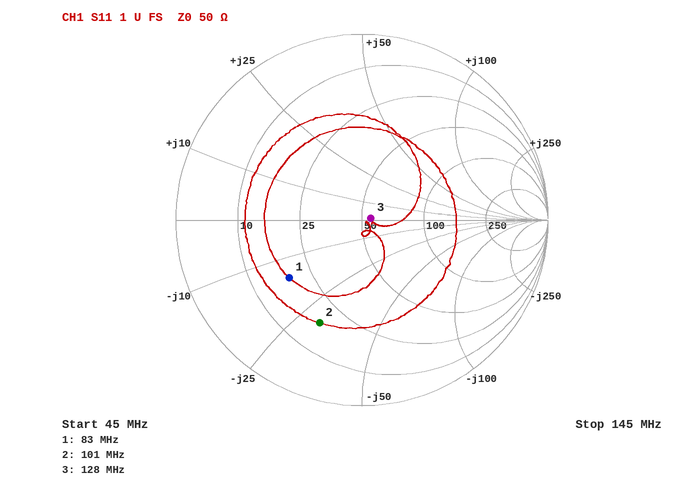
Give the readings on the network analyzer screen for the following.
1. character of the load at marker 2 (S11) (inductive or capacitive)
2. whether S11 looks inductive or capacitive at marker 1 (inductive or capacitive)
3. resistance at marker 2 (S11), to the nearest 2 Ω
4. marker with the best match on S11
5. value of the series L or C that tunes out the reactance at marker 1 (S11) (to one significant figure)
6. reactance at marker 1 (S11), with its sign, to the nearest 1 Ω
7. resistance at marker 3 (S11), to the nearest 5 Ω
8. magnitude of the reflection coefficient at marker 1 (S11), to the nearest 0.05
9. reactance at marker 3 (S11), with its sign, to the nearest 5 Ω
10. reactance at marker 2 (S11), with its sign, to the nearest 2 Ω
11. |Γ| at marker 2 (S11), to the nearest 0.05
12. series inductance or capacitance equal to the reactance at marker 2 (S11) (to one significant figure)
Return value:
capacitive
capacitive
18 Ω
marker 3
30 nH
-15 Ω
55 Ω
0.50
0 Ω
-30 Ω
0.60
50 pF
